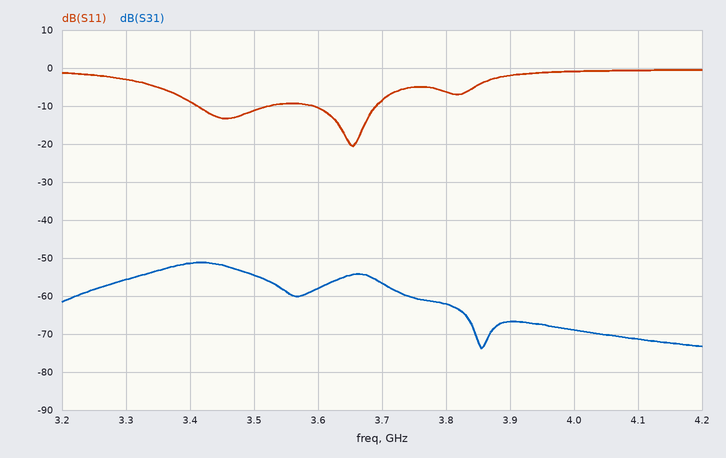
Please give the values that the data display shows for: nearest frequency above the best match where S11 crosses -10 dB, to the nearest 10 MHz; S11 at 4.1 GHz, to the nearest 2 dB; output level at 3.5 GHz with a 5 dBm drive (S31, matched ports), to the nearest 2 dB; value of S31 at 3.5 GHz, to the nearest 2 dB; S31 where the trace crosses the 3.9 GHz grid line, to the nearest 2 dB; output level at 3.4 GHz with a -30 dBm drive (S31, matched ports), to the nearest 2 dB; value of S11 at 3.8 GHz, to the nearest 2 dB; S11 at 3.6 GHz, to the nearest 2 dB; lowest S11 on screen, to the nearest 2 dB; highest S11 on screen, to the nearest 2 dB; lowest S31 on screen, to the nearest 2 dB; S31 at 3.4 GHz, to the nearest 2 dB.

3.69 GHz
0 dB
-50 dBm
-54 dB
-66 dB
-82 dBm
-6 dB
-10 dB
-20 dB
0 dB
-74 dB
-52 dB
